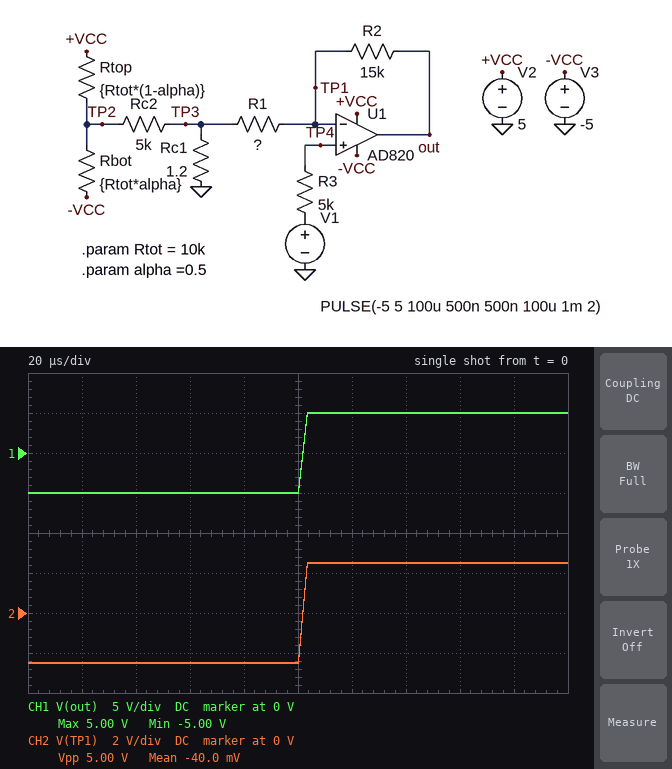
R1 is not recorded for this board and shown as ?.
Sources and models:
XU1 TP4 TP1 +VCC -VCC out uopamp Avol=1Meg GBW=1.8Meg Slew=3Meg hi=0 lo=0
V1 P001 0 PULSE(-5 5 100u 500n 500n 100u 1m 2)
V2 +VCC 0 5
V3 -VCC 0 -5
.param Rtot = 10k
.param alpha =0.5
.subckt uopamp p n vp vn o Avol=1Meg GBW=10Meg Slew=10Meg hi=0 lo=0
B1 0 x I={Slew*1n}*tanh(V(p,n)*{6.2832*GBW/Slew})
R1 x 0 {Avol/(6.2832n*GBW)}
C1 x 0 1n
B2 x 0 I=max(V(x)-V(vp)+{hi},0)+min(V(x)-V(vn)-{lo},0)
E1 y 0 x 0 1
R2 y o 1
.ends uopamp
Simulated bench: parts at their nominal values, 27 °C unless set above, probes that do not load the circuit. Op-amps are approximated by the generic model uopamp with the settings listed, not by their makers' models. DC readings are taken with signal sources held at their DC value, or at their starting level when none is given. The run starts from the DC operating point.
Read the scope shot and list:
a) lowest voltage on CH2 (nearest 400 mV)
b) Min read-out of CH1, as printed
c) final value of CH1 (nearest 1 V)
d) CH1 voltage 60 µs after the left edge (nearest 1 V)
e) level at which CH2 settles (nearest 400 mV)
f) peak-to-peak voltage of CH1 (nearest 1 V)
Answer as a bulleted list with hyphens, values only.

- -2.4 V
- -5.00 V
- 5 V
- -5 V
- 2.4 V
- 10 V
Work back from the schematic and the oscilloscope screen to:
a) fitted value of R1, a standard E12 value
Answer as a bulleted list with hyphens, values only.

- 15 kΩ
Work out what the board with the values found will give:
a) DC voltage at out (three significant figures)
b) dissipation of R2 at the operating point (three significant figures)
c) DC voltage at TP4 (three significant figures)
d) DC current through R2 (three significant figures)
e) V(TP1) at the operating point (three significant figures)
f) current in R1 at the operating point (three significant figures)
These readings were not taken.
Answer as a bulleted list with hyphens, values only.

- -5.00 V
- 417 µW
- -5.00 V
- 167 µA
- -2.50 V
- 167 µA
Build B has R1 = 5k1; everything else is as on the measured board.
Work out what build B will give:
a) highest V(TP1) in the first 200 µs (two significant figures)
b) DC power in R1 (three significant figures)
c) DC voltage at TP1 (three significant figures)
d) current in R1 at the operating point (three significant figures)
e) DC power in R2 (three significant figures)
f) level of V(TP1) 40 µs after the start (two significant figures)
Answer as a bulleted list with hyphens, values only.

- 1.3 V
- 316 µW
- -1.27 V
- 249 µA
- 929 µW
- -1.3 V
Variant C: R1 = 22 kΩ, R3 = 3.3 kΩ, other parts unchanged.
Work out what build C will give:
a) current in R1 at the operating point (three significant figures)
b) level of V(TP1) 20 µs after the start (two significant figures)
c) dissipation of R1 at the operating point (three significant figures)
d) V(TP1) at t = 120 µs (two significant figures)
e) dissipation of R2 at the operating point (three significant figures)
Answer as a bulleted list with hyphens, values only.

- 135 µA
- -3.0 V
- 402 µW
- 3.0 V
- 274 µW
